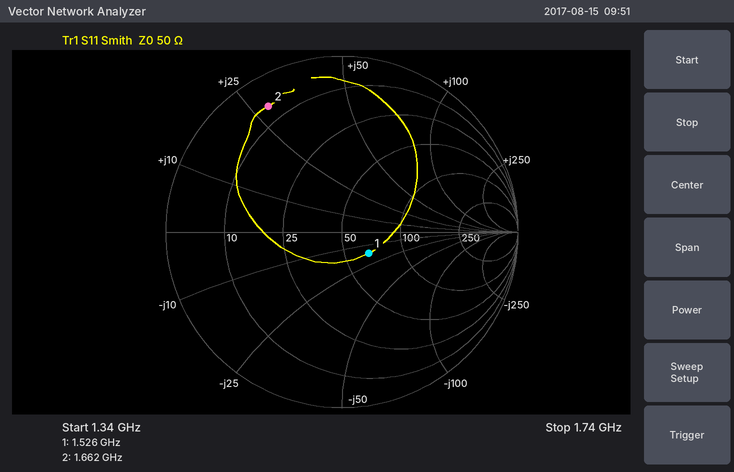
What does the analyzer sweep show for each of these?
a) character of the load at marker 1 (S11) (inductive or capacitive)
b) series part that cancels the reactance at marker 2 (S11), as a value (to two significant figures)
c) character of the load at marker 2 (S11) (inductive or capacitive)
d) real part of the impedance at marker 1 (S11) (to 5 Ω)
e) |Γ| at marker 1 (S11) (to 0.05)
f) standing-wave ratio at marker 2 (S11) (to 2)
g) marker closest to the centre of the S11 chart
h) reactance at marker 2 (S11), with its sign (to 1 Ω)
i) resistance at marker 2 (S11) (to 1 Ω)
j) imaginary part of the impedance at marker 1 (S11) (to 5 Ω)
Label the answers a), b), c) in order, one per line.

a) capacitive
b) 3.4 pF
c) inductive
d) 65 Ω
e) 0.20
f) 10
g) marker 1
h) +28 Ω
i) 6 Ω
j) -15 Ω
